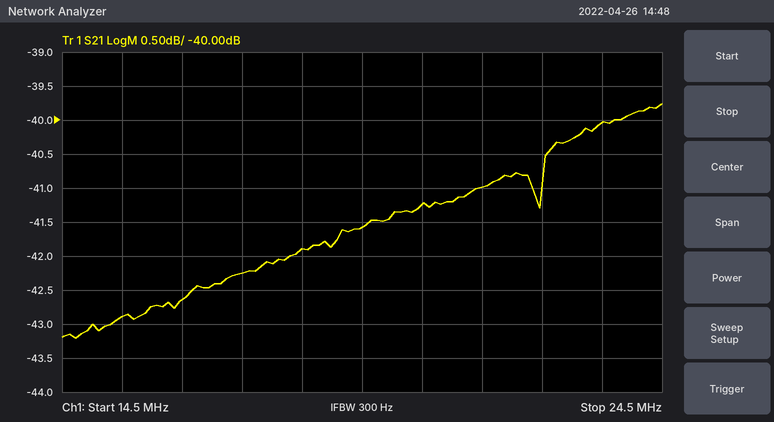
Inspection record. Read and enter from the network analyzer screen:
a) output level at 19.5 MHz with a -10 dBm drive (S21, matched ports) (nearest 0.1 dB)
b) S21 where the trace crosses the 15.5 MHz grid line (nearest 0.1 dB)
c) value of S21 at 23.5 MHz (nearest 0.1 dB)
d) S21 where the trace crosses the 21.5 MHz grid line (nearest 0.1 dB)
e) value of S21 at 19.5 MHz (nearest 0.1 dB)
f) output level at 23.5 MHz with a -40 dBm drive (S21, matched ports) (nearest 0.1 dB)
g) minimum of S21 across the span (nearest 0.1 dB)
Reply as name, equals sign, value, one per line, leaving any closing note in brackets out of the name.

output level at 19.5 MHz with a -10 dBm drive (S21, matched ports) = -51.6 dBm
S21 where the trace crosses the 15.5 MHz grid line = -42.9 dB
value of S21 at 23.5 MHz = -40.0 dB
S21 where the trace crosses the 21.5 MHz grid line = -41.0 dB
value of S21 at 19.5 MHz = -41.6 dB
output level at 23.5 MHz with a -40 dBm drive (S21, matched ports) = -80.0 dBm
minimum of S21 across the span = -43.2 dB
